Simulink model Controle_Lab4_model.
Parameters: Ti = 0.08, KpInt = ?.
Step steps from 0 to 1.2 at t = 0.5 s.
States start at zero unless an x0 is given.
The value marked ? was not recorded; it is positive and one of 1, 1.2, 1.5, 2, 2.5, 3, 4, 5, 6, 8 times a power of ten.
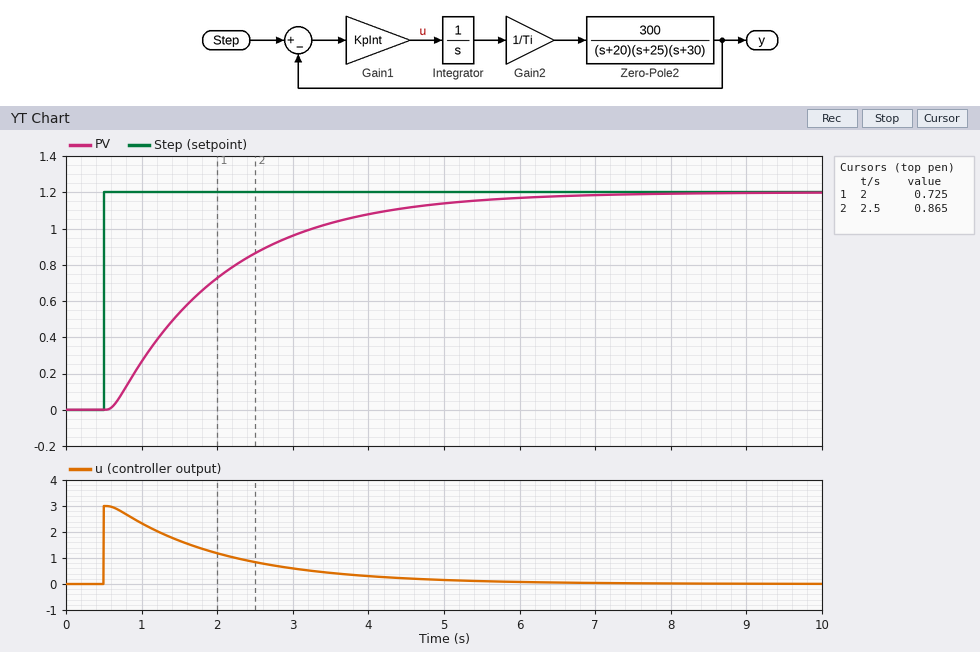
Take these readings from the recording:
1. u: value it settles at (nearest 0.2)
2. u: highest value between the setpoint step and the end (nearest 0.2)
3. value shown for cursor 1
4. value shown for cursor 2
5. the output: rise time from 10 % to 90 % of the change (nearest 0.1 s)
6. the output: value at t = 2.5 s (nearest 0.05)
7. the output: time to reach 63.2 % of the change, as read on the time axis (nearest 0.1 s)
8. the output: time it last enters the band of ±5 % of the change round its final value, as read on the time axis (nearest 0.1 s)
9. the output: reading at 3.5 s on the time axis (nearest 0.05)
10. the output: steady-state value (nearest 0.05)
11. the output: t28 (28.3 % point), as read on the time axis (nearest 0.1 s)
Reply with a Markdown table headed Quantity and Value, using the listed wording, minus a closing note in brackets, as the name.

| Quantity | Value |
|---|---|
| u: value it settles at | 0.0 |
| u: highest value between the setpoint step and the end | 3.0 |
| value shown for cursor 1 | 0.725 |
| value shown for cursor 2 | 0.865 |
| the output: rise time from 10 % to 90 % of the change | 3.2 s |
| the output: value at t = 2.5 s | 0.85 |
| the output: time to reach 63.2 % of the change, as read on the time axis | 2.1 s |
| the output: time it last enters the band of ±5 % of the change round its final value, as read on the time axis | 5.0 s |
| the output: reading at 3.5 s on the time axis | 1.05 |
| the output: steady-state value | 1.20 |
| the output: t28 (28.3 % point), as read on the time axis | 1.1 s |
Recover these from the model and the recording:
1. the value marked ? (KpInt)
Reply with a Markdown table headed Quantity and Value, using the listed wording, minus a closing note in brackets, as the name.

| Quantity | Value |
|---|---|
| the value marked ? | 2.5 |
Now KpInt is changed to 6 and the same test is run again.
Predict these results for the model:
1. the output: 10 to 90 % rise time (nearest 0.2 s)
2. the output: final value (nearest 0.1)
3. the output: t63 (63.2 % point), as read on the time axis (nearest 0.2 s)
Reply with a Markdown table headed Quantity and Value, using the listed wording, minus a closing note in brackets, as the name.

| Quantity | Value |
|---|---|
| the output: 10 to 90 % rise time | 1.2 s |
| the output: final value | 1.2 |
| the output: t63 (63.2 % point), as read on the time axis | 1.2 s |
